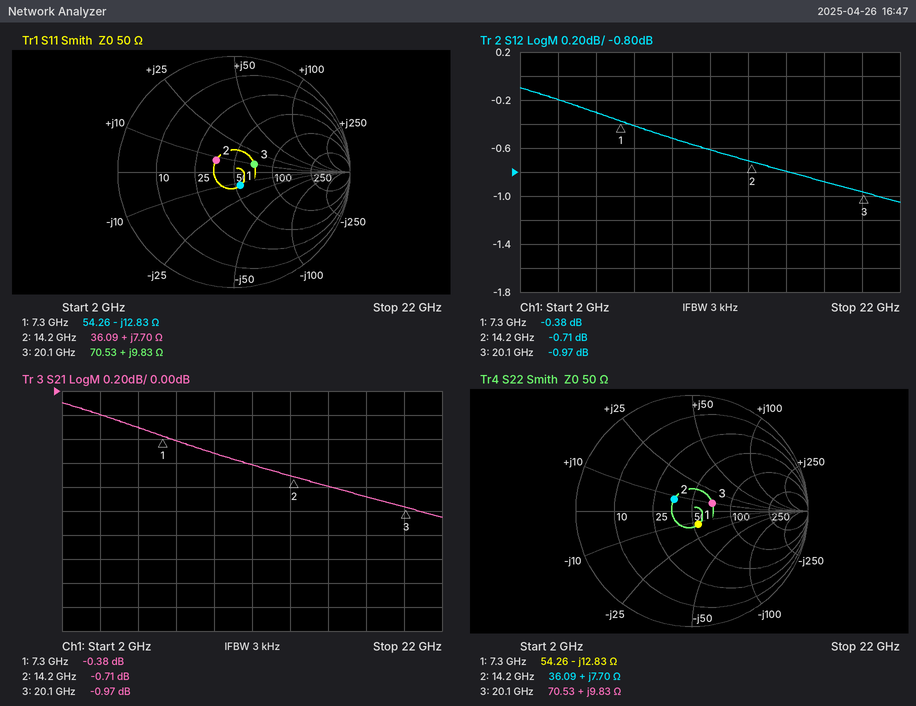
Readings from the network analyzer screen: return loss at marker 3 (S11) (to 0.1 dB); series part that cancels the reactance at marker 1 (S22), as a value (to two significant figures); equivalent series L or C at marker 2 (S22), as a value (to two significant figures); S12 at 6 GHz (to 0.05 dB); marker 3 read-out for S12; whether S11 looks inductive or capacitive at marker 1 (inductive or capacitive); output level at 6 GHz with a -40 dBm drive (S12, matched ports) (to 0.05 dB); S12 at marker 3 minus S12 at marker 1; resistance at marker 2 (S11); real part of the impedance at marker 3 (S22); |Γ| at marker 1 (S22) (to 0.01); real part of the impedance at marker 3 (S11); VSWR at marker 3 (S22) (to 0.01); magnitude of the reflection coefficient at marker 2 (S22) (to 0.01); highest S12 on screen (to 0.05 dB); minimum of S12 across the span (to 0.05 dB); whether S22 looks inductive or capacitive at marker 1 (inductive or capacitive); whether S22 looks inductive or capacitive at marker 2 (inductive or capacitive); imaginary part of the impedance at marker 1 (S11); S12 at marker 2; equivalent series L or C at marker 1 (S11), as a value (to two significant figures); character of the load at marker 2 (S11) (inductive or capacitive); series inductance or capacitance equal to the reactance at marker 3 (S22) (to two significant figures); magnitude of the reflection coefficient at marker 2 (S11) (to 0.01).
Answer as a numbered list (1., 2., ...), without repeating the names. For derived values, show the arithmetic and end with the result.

1. 14.5 dB
2. L = 12.83 Ω/(2π × 7.3 GHz) ≈ 280 pH
3. L = 7.7 Ω/(2π × 14.2 GHz) ≈ 86 pH
4. -0.30 dB
5. -0.97 dB
6. capacitive
7. -40 dBm + (-0.30 dB) = -40.30 dBm
8. -0.97 − (-0.38) = -0.59 dB
9. 36.09 Ω
10. 70.53 Ω
11. 0.13
12. 70.53 Ω
13. 1.46
14. 0.18
15. -0.10 dB
16. -1.05 dB
17. capacitive
18. inductive
19. -12.83 Ω
20. -0.71 dB
21. C = 1/(2π × 7.3 GHz × 12.83 Ω) ≈ 1.7 pF
22. inductive
23. L = 9.83 Ω/(2π × 20.1 GHz) ≈ 78 pH
24. 0.18
